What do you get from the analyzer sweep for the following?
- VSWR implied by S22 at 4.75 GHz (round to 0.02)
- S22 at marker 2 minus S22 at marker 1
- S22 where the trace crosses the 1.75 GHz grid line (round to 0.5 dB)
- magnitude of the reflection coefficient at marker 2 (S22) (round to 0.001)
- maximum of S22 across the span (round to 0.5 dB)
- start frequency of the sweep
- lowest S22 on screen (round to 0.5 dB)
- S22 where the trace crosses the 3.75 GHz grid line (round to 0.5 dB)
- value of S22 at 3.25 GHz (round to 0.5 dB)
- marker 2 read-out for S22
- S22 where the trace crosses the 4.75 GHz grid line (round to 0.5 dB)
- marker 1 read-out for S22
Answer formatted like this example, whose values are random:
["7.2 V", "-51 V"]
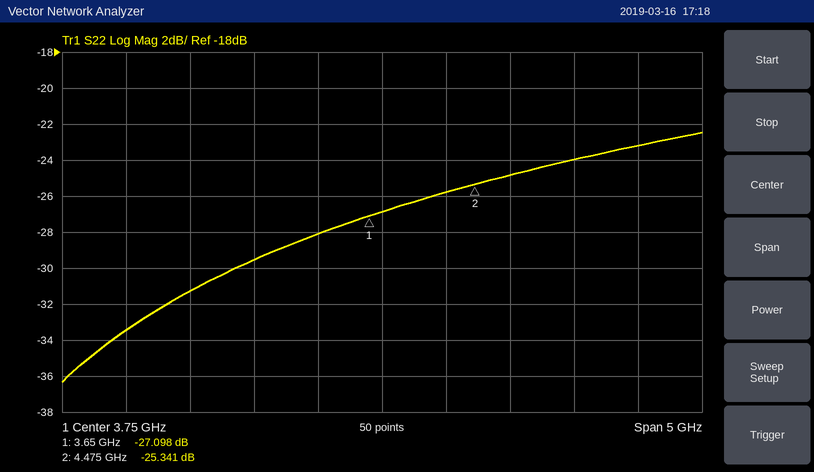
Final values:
["1.12", "1.757 dB", "-33.5 dB", "0.054", "-22.5 dB", "1.25 GHz", "-36.5 dB", "-27.0 dB", "-28.0 dB", "-25.341 dB", "-25.0 dB", "-27.098 dB"]
